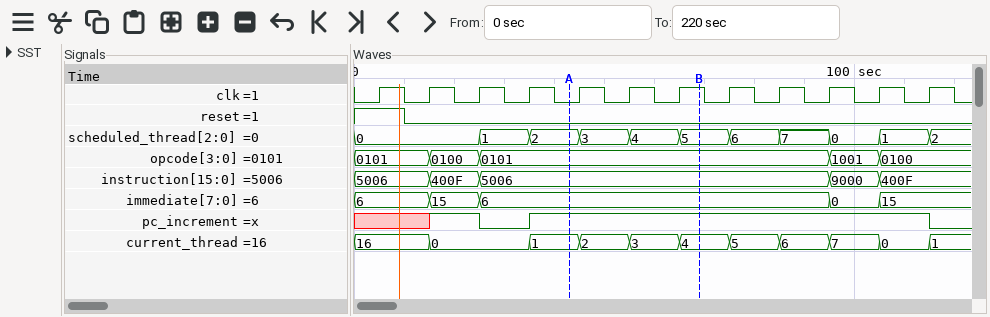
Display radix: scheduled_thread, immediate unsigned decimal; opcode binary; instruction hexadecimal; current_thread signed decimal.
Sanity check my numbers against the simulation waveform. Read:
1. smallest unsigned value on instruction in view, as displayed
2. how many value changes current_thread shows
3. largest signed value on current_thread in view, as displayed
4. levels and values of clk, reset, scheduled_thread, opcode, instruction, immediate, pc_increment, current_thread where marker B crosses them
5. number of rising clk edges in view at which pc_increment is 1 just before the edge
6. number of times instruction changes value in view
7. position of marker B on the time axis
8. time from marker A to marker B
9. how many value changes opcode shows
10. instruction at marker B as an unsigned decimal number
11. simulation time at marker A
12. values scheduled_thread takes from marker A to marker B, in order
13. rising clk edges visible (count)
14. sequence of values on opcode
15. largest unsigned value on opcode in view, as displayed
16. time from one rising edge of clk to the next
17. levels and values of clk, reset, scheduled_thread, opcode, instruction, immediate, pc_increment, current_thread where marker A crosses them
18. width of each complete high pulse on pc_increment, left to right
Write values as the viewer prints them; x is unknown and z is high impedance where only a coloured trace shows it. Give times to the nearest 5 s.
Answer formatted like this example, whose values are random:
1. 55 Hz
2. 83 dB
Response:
1. 400F
2. 10
3. 16
4. clk=1, reset=0, scheduled_thread=5, opcode=0101, instruction=5006, immediate=6, pc_increment=1, current_thread=4
5. 9
6. 4
7. 70 s
8. 25 s
9. 4
10. 20486
11. 45 s
12. 2, 3, 4, 5
13. 12
14. 0101, 0100, 0101, 1001, 0100
15. 1001
16. 10 s
17. clk=0, reset=0, scheduled_thread=2, opcode=0101, instruction=5006, immediate=6, pc_increment=1, current_thread=1
18. 80 s
